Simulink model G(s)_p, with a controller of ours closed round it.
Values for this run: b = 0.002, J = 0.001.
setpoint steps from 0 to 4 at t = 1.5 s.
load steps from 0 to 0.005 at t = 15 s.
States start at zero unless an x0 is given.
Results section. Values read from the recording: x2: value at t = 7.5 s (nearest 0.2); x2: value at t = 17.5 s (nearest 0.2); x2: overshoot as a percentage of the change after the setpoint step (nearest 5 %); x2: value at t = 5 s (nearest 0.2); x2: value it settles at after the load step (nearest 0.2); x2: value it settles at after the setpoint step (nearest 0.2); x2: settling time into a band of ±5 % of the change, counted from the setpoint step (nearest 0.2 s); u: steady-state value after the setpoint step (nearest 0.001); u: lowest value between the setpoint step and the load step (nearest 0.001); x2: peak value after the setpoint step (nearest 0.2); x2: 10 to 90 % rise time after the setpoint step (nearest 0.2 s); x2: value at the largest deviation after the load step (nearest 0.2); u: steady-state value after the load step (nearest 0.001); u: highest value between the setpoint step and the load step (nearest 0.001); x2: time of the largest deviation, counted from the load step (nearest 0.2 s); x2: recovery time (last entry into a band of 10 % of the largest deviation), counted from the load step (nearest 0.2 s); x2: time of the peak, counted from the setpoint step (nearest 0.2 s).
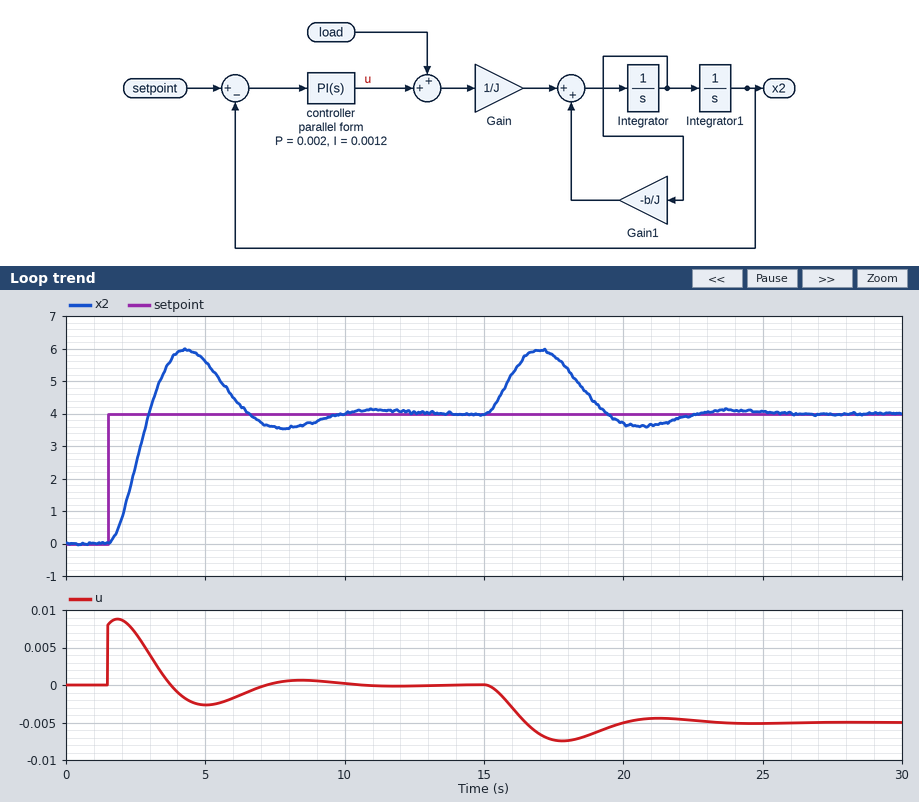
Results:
3.6
5.8
50 %
5.6
4.0
4.0
7.6 s
0.000
-0.003
6.0
1.0 s
6.0
-0.005
0.009
2.0 s
6.8 s
2.8 s
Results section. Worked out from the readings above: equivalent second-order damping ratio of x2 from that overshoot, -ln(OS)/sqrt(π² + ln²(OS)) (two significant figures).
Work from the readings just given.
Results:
0.22
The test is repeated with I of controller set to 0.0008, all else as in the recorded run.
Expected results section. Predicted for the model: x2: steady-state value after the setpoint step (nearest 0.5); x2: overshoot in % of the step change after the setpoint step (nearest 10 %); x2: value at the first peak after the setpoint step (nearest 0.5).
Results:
4.0
40 %
5.5
